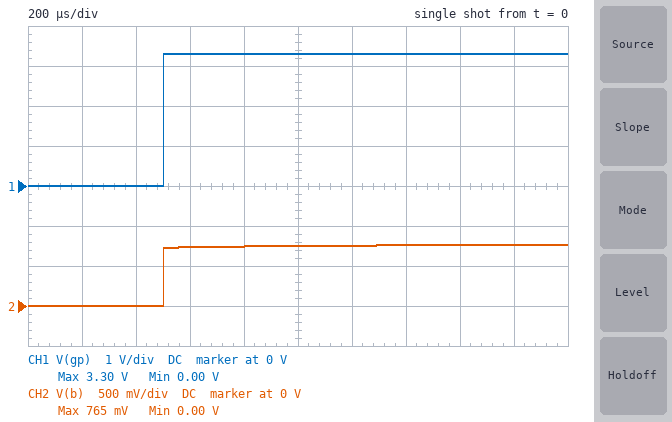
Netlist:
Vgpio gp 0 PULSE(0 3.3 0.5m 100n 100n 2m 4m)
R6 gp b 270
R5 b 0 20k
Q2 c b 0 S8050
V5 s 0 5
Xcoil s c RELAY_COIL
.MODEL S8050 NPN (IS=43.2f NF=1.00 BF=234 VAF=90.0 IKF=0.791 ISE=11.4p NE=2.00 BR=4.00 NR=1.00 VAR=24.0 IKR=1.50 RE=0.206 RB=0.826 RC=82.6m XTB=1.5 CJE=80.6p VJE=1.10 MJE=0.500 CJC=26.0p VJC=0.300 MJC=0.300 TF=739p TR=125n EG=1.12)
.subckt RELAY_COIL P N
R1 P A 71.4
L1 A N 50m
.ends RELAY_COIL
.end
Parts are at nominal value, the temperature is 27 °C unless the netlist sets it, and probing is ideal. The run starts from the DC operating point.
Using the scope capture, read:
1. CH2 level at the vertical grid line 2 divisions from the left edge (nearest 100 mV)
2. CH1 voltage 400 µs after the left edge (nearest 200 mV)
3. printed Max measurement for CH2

0 V
0 V
765 mV
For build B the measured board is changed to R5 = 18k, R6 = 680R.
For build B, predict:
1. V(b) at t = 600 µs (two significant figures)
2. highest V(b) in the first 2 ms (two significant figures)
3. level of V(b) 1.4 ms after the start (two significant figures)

710 mV
750 mV
740 mV
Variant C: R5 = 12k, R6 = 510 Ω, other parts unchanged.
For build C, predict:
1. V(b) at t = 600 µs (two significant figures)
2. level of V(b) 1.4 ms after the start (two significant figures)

720 mV
750 mV
